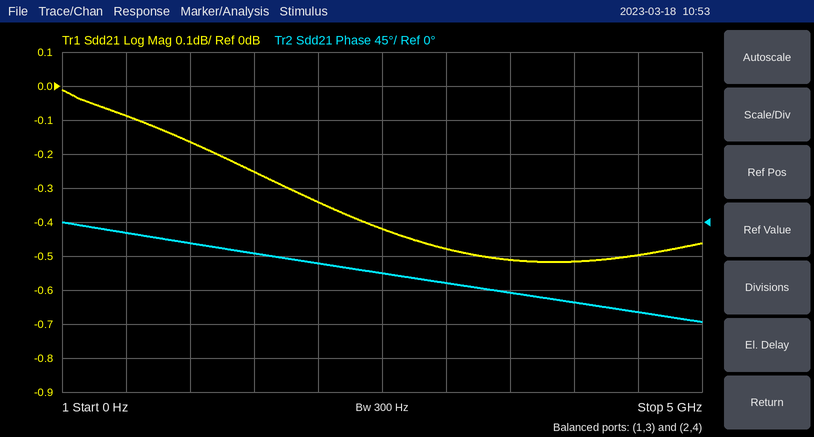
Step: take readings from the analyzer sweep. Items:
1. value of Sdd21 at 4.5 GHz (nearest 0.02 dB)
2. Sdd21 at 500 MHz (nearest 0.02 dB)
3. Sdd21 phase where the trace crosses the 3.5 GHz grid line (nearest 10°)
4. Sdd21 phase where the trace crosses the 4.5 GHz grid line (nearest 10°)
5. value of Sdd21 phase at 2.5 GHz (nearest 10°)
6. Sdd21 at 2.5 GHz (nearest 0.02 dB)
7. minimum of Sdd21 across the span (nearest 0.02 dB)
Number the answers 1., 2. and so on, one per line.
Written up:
1. -0.50 dB
2. -0.08 dB
3. -90°
4. -120°
5. -70°
6. -0.42 dB
7. -0.52 dB
